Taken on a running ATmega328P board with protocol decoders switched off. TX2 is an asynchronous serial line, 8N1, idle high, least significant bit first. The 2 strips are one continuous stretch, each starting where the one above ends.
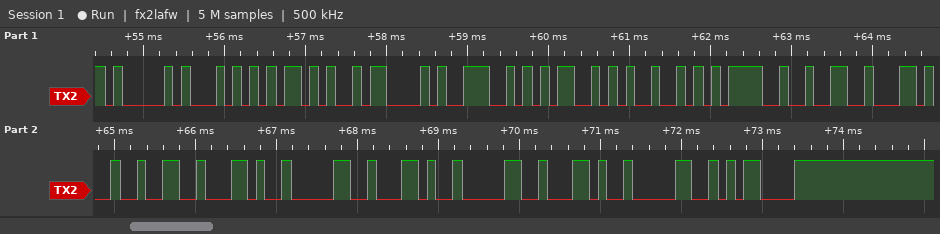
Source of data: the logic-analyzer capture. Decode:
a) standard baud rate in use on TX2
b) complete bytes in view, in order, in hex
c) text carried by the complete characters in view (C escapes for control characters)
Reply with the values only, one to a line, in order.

9600 baud
0x41 0x54 0x2B 0x43 0x4E 0x4D 0x49 0x3D 0x32 0x2C 0x32 0x2C 0x30 0x2C 0x30 0x2C 0x30 0x0D
"AT+CNMI=2,2,0,0,0\r"
